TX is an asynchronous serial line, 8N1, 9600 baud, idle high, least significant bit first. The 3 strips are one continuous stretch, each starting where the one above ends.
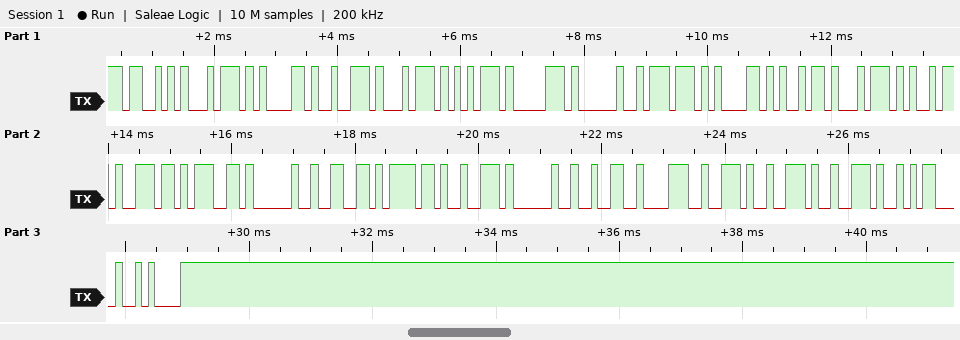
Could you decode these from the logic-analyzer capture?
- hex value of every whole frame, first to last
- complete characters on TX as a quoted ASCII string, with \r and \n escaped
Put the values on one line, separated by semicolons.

53 74 61 72 74 75 70 20 77 61 69 74 69 6E 67 20 66 6F 72 20 32 38 2E 2E 2E 0D 0A; "Startup waiting for 28...\r\n"
